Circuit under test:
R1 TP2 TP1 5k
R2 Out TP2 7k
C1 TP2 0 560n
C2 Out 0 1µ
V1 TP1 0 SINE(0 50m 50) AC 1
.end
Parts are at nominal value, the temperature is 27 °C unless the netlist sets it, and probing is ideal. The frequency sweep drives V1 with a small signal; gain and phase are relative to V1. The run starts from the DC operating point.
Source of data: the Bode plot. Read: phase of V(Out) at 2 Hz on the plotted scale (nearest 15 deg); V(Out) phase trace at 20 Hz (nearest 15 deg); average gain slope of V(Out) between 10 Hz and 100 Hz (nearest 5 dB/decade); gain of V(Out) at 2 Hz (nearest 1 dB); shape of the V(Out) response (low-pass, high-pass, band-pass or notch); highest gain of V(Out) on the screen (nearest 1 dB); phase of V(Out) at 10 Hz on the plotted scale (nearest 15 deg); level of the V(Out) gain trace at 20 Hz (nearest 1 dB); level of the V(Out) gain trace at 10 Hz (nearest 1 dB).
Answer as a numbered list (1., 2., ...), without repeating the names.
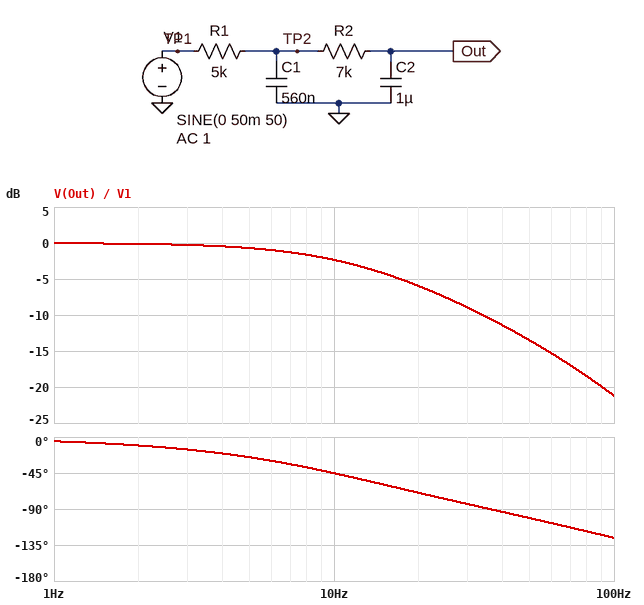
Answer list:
1. -15 deg
2. -75 deg
3. -20 dB/decade
4. 0 dB
5. low-pass
6. 0 dB
7. -45 deg
8. -6 dB
9. -2 dB
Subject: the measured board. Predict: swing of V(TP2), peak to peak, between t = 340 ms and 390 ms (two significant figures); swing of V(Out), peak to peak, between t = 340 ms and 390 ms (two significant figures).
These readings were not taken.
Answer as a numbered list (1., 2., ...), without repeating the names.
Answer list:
1. 51 mV
2. 21 mV
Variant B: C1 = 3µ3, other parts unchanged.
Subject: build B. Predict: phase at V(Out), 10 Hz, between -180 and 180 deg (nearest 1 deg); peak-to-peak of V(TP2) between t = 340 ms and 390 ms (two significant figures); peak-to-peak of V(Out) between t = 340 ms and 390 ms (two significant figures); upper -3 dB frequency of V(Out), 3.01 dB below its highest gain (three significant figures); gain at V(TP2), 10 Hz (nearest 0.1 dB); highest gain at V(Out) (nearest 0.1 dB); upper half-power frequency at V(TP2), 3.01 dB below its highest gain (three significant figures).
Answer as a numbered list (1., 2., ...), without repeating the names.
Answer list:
1. -73 deg
2. 18 mV
3. 7.3 mV
4. 6.48 Hz
5. -4.7 dB
6. 0 dB
7. 7.05 Hz
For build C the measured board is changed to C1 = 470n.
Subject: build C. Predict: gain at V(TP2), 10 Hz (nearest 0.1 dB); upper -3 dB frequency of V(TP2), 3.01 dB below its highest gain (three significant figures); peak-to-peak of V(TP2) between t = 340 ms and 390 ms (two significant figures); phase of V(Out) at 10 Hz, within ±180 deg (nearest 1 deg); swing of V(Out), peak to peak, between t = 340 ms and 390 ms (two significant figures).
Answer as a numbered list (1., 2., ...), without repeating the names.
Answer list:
1. -1.5 dB
2. 18.0 Hz
3. 53 mV
4. -44 deg
5. 22 mV
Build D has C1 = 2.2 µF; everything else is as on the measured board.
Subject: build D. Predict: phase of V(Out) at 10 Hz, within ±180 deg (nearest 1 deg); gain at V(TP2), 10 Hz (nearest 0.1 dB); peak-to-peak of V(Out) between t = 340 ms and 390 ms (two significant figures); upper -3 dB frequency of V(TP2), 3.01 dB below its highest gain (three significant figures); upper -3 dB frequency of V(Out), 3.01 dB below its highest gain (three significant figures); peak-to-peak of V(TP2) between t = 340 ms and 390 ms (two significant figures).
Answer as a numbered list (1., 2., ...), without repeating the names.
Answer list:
1. -64 deg
2. -3.3 dB
3. 10 mV
4. 9.24 Hz
5. 8.06 Hz
6. 25 mV
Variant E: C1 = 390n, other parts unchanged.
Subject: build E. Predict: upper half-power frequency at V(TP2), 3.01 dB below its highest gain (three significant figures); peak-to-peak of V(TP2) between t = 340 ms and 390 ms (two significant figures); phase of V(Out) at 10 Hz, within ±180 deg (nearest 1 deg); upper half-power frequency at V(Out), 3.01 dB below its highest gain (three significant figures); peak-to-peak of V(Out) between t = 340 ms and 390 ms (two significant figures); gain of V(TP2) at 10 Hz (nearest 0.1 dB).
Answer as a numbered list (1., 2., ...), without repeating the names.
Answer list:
1. 18.8 Hz
2. 55 mV
3. -43 deg
4. 12.3 Hz
5. 23 mV
6. -1.4 dB
